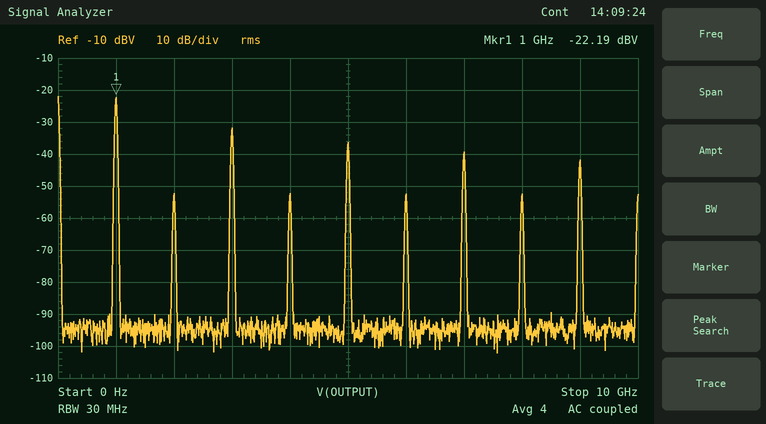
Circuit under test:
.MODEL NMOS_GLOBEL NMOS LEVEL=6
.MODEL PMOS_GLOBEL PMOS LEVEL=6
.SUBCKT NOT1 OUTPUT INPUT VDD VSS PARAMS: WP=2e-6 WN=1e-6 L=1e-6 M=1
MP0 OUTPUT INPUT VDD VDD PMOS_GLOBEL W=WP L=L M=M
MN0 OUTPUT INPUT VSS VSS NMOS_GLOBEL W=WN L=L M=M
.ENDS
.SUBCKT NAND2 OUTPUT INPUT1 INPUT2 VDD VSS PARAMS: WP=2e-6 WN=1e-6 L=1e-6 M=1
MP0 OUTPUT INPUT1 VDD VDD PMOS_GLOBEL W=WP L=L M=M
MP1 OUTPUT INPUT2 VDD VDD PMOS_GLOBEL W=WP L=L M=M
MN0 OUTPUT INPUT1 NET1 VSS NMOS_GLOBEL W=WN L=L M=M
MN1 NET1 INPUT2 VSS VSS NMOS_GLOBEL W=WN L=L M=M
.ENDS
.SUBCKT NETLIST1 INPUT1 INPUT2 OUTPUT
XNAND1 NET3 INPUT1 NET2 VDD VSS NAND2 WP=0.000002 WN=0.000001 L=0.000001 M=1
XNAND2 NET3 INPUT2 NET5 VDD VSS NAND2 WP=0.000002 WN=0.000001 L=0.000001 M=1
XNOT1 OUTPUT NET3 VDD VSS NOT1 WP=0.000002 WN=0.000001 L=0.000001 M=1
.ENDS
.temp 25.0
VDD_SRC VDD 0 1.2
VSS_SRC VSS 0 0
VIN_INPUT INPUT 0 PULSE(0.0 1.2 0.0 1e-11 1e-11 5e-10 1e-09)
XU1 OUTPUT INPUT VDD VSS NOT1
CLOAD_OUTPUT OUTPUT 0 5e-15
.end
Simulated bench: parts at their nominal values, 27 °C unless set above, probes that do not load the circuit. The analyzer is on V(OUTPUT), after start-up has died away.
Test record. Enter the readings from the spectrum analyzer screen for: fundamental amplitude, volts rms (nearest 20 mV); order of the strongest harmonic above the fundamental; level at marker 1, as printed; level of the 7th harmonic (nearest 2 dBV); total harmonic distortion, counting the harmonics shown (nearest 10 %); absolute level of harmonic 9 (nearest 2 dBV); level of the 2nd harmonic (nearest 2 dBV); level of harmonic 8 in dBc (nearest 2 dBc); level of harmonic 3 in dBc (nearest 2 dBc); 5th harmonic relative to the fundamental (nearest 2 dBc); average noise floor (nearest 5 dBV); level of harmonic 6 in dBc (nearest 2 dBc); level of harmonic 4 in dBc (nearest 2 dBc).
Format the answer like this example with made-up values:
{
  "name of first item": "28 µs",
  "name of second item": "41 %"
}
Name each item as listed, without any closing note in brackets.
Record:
{
  "fundamental amplitude, volts rms": "80 mV",
  "order of the strongest harmonic above the fundamental": "3",
  "level at marker 1, as printed": "-22.19 dBV",
  "level of the 7th harmonic": "-40 dBV",
  "total harmonic distortion, counting the harmonics shown": "40 %",
  "absolute level of harmonic 9": "-42 dBV",
  "level of the 2nd harmonic": "-52 dBV",
  "level of harmonic 8 in dBc": "-30 dBc",
  "level of harmonic 3 in dBc": "-10 dBc",
  "5th harmonic relative to the fundamental": "-14 dBc",
  "average noise floor": "-95 dBV",
  "level of harmonic 6 in dBc": "-30 dBc",
  "level of harmonic 4 in dBc": "-30 dBc"
}
